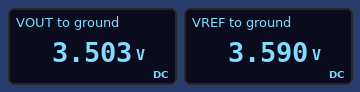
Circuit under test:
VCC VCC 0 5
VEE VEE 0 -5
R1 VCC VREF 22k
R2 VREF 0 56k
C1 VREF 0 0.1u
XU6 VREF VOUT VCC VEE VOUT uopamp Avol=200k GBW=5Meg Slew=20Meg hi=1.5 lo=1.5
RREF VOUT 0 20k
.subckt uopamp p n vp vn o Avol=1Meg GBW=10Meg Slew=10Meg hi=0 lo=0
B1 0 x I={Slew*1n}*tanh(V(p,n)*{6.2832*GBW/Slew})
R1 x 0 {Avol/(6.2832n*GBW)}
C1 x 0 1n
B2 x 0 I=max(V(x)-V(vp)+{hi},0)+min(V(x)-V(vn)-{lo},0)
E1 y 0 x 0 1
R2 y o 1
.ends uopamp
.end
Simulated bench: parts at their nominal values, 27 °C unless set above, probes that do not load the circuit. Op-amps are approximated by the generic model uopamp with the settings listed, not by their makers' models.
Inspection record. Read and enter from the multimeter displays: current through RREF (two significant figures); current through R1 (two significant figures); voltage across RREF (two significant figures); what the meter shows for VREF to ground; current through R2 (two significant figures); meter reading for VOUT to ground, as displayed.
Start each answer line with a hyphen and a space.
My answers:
- 180 µA
- 64 µA
- 3.5 V
- 3.590 V
- 64 µA
- 3.503 V
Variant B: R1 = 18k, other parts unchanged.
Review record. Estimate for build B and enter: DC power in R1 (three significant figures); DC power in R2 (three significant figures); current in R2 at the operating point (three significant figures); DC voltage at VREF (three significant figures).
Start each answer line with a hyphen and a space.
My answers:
- 82.2 µW
- 256 µW
- 67.6 µA
- 3.78 V
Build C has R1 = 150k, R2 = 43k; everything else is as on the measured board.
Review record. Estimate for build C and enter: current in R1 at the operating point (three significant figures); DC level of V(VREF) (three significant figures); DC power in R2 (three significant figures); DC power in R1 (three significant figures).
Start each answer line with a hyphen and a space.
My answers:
- 25.9 µA
- 1.11 V
- 28.9 µW
- 101 µW
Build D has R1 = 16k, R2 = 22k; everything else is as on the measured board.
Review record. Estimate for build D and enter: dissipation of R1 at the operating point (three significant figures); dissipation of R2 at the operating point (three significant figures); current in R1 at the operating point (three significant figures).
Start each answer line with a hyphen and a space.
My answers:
- 277 µW
- 381 µW
- 132 µA
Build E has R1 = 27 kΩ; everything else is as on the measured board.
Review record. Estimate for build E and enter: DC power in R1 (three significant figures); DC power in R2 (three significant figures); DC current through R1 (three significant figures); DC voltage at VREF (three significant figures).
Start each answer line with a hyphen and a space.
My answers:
- 98.0 µW
- 203 µW
- 60.2 µA
- 3.37 V
